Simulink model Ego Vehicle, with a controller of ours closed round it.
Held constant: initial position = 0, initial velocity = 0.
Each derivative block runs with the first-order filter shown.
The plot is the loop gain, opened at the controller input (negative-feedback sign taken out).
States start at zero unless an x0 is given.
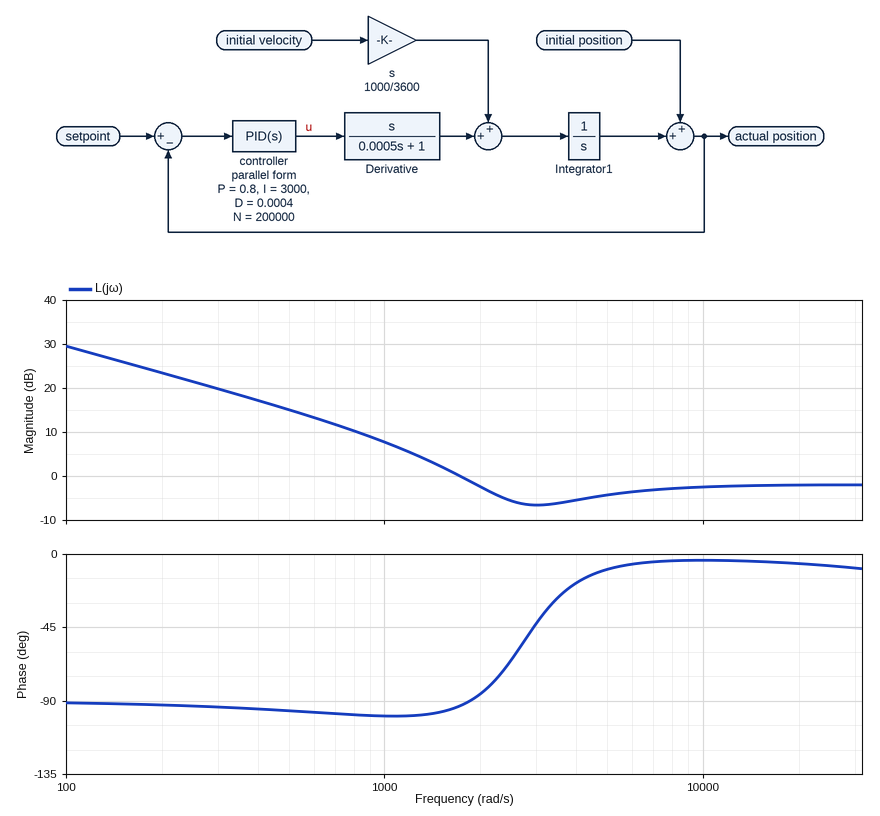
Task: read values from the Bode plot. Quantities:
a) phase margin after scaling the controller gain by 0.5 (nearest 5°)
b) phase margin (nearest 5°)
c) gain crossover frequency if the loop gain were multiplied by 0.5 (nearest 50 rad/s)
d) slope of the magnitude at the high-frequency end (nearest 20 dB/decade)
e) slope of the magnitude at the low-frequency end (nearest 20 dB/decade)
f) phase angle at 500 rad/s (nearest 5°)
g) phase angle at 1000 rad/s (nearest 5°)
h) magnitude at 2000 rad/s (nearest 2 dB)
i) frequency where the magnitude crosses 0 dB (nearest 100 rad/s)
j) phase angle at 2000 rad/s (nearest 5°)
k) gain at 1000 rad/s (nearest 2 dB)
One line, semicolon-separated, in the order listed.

80°; 85°; 1150 rad/s; 0 dB/decade; -20 dB/decade; -95°; -100°; -2 dB; 1700 rad/s; -85°; 8 dB
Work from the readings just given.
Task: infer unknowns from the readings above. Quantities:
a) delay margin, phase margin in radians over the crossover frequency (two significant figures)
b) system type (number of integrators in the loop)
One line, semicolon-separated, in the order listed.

0.00087 s; 1
